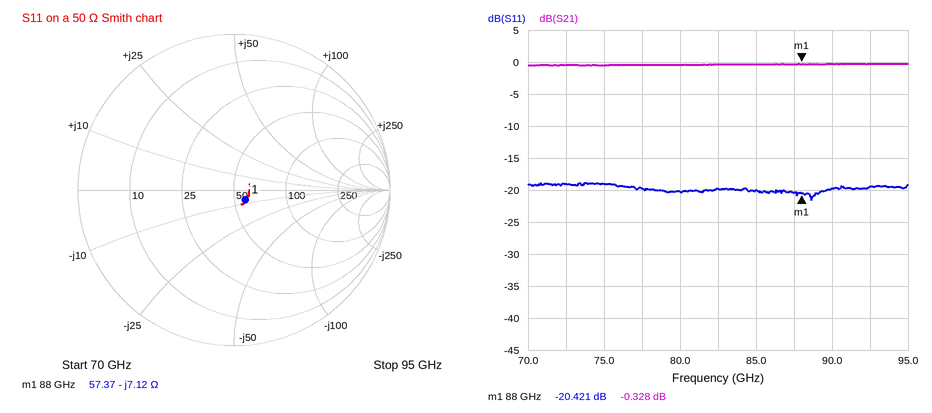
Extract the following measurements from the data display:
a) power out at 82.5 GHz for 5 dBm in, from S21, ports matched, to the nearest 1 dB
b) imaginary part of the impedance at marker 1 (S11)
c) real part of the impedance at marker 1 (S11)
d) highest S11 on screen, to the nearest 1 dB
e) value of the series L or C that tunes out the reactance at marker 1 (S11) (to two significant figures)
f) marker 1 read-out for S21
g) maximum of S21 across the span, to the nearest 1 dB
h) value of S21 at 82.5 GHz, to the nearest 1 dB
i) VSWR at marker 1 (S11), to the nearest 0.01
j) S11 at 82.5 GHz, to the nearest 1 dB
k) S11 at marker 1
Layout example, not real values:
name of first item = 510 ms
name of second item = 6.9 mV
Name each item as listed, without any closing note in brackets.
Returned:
power out at 82.5 GHz for 5 dBm in, from S21, ports matched, to the nearest 1 dB = 5 dBm
imaginary part of the impedance at marker 1 = -7.12 Ω
real part of the impedance at marker 1 = 57.37 Ω
highest S11 on screen, to the nearest 1 dB = -19 dB
value of the series L or C that tunes out the reactance at marker 1 (S11) = 13 pH
marker 1 read-out for S21 = -0.328 dB
maximum of S21 across the span, to the nearest 1 dB = 0 dB
value of S21 at 82.5 GHz, to the nearest 1 dB = 0 dB
VSWR at marker 1 (S11), to the nearest 0.01 = 1.21
S11 at 82.5 GHz, to the nearest 1 dB = -20 dB
S11 at marker 1 = -20.421 dB
